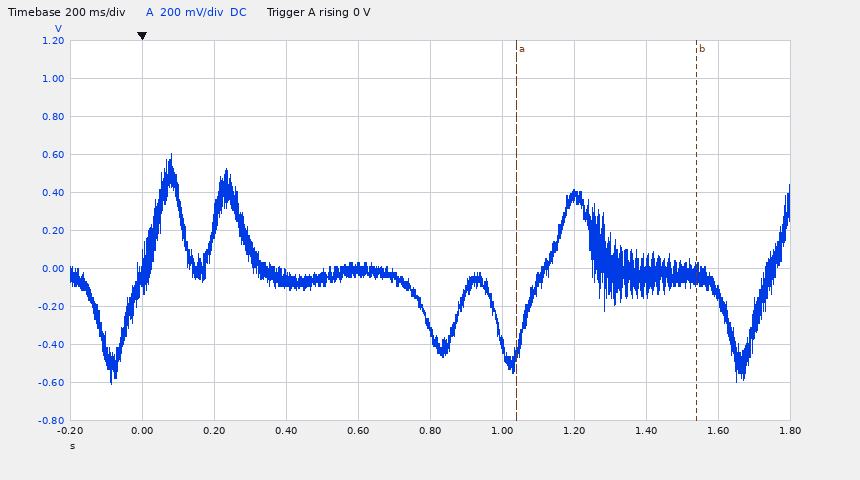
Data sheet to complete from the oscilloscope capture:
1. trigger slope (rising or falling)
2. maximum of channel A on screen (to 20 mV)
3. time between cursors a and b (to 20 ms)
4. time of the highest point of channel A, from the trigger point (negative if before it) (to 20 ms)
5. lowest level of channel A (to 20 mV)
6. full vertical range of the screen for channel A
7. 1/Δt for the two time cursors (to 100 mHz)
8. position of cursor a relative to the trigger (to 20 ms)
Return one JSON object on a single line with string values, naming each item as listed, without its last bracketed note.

{"trigger slope": "rising", "maximum of channel A on screen": "600 mV", "time between cursors a and b": "500 ms", "time of the highest point of channel A, from the trigger point (negative if before it)": "+80 ms", "lowest level of channel A": "-600 mV", "full vertical range of the screen for channel A": "2 V", "1/Δt for the two time cursors": "2.0 Hz", "position of cursor a relative to the trigger": "+1.04 s"}
